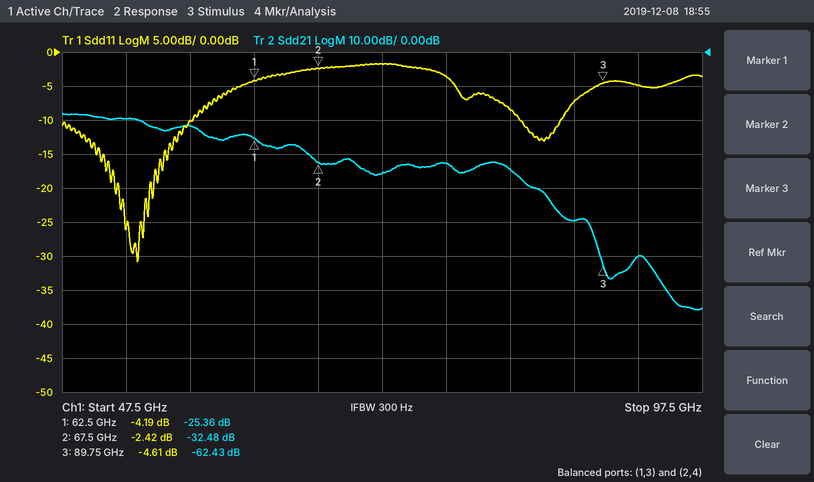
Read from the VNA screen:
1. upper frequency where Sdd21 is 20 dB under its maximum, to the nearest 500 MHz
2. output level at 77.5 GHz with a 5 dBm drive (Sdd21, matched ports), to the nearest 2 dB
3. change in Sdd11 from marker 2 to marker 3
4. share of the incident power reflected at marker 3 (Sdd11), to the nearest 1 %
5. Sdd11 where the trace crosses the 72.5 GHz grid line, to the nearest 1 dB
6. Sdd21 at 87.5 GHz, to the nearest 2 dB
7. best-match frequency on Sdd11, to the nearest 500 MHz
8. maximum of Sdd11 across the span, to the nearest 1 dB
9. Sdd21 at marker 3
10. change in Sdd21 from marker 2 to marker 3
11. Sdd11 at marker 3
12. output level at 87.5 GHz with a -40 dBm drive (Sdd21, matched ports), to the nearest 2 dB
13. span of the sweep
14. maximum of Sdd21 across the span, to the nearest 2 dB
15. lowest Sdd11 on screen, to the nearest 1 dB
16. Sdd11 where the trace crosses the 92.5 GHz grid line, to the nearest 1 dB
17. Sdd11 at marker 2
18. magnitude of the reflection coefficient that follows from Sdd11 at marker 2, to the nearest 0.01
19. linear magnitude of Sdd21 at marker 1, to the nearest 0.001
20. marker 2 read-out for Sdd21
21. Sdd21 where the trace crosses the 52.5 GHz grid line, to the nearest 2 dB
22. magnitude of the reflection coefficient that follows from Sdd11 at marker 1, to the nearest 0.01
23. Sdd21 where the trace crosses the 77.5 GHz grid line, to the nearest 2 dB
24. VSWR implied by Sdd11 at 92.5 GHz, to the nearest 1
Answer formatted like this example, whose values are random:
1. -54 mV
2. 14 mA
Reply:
1. 83.5 GHz
2. -28 dBm
3. -2.19 dB
4. 35 %
5. -2 dB
6. -50 dB
7. 53.5 GHz
8. -2 dB
9. -62.43 dB
10. -29.95 dB
11. -4.61 dB
12. -90 dBm
13. 50 GHz
14. -18 dB
15. -31 dB
16. -5 dB
17. -2.42 dB
18. 0.76
19. 0.054
20. -32.48 dB
21. -20 dB
22. 0.62
23. -32 dB
24. 4
